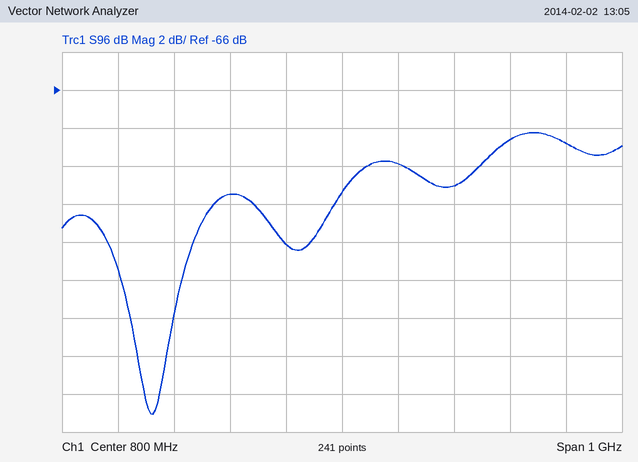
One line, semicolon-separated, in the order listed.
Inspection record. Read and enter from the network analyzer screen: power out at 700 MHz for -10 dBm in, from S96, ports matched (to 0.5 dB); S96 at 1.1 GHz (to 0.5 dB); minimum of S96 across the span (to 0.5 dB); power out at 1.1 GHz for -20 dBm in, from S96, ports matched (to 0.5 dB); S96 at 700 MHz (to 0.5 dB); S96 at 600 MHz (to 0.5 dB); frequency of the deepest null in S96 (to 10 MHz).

-84.0 dBm; -68.5 dB; -83.0 dB; -88.5 dBm; -74.0 dB; -71.5 dB; 460 MHz
